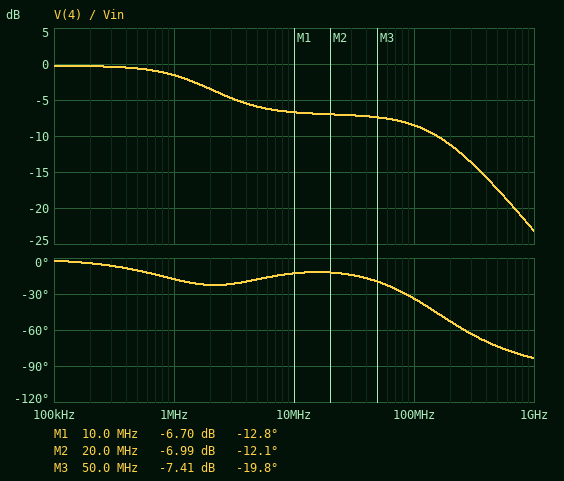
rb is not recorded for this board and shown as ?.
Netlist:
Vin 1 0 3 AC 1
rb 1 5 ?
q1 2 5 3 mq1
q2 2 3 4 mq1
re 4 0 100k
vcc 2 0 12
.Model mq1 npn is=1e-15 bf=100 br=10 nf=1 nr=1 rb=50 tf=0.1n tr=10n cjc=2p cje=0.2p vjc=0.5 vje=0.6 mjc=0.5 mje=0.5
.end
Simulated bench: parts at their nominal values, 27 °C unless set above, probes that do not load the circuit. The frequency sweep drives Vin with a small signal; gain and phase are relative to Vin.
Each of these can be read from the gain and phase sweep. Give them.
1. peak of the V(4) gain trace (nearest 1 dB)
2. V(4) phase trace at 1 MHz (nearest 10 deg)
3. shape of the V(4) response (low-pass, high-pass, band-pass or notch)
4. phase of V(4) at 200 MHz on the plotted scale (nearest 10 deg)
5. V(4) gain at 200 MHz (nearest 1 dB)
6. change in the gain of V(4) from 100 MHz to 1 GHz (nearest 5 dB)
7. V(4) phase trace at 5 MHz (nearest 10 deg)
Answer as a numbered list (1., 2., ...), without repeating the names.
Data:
1. 0 dB
2. -20 deg
3. low-pass
4. -50 deg
5. -11 dB
6. -15 dB
7. -20 deg
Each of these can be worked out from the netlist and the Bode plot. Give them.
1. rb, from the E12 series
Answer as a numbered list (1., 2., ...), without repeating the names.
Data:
1. 1.5 kΩ
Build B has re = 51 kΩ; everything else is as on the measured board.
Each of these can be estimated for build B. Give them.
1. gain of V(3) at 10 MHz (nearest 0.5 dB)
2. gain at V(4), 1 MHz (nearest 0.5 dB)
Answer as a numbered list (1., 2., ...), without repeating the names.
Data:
1. -6.0 dB
2. -0.5 dB
